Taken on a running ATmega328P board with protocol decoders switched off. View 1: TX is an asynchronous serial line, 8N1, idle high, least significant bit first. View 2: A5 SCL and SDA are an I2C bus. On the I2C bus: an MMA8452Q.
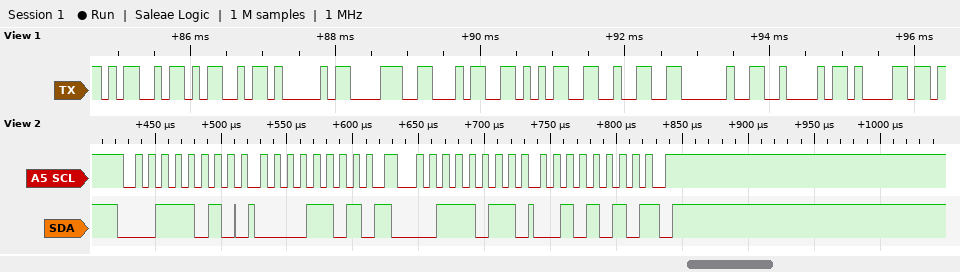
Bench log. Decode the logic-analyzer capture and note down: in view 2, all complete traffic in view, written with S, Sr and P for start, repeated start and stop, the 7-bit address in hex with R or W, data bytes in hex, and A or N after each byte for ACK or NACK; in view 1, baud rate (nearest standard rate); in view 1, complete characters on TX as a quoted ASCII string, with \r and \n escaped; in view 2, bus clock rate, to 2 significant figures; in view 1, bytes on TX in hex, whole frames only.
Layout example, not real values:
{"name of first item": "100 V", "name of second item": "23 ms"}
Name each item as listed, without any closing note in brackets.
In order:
{"in view 2, all complete traffic in view, written with S, Sr and P for start, repeated start and stop, the 7-bit address in hex with R or W, data bytes in hex, and A or N after each byte for ACK or NACK": "S 1DW A 0D A Sr 1DR A 2A N P", "in view 1, baud rate": "9600 baud", "in view 1, complete characters on TX as a quoted ASCII string, with \\r and \\n escaped": "\"MMA8452 Ba\"", "in view 2, bus clock rate, to 2 significant figures": "100 kHz", "in view 1, bytes on TX in hex, whole frames only": "4D 4D 41 38 34 35 32 20 42 61"}
